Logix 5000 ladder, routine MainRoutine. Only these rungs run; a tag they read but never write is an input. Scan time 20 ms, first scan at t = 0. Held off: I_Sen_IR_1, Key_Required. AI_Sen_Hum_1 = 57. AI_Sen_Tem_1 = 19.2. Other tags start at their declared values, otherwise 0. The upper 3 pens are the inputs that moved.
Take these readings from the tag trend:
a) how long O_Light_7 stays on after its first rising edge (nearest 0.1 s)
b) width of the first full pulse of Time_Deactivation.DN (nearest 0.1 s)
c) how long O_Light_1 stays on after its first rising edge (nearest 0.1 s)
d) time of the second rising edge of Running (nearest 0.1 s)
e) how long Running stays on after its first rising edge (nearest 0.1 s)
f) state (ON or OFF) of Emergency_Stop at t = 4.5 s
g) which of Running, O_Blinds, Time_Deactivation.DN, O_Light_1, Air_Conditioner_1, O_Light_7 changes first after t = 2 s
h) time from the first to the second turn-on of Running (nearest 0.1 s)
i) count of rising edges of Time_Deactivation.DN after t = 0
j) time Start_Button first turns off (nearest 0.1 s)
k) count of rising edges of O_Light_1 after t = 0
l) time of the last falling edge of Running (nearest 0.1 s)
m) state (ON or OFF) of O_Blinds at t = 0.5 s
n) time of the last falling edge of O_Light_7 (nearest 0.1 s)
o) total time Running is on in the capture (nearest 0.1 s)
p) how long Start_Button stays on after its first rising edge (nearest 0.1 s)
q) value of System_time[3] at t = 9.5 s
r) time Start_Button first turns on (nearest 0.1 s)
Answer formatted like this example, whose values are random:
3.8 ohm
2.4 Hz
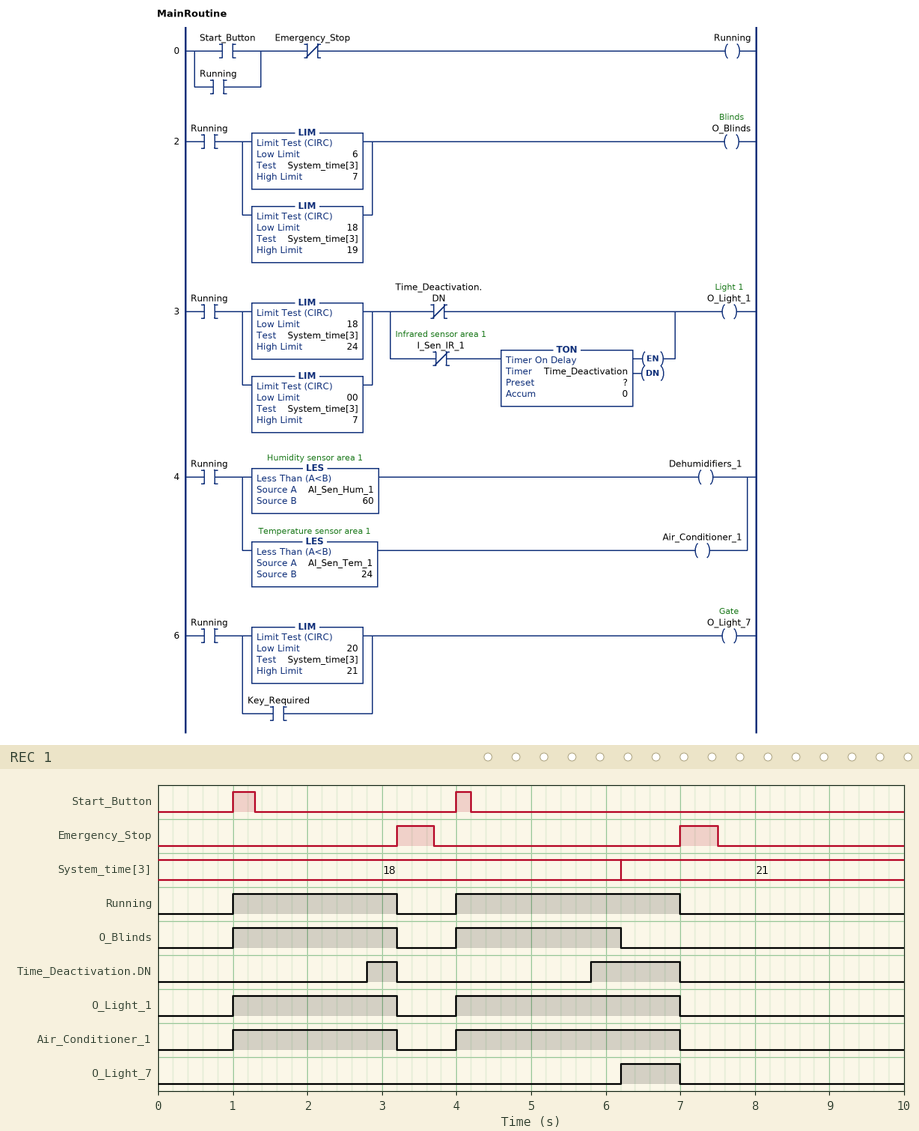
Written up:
0.8 s
0.4 s
2.2 s
4.0 s
2.2 s
OFF
Time_Deactivation.DN
3.0 s
2
1.3 s
2
7.0 s
OFF
7.0 s
5.2 s
0.3 s
21
1.0 s
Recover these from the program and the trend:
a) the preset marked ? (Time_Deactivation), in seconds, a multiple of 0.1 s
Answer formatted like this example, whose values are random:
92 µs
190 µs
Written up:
1.8 s
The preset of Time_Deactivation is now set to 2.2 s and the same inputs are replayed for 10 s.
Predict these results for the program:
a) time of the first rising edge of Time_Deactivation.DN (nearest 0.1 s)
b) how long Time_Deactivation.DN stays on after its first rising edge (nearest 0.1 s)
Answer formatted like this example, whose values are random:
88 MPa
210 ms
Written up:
6.2 s
0.8 s
